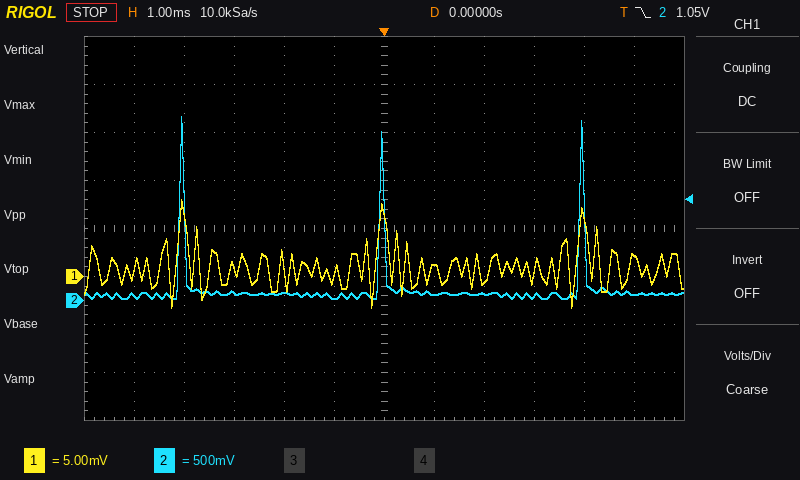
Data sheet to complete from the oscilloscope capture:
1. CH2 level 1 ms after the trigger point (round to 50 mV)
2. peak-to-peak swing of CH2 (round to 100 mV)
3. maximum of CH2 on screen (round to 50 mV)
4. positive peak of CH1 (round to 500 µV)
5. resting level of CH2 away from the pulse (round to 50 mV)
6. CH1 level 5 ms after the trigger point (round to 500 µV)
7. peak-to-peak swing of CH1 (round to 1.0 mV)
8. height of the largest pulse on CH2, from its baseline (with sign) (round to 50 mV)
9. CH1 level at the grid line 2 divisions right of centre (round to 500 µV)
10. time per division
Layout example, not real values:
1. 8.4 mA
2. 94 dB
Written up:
1. 50 mV
2. 1.90 V
3. 1.90 V
4. 8.0 mV
5. 50 mV
6. 2.0 mV
7. 11.0 mV
8. +1.85 V
9. -500 µV
10. 1 ms
